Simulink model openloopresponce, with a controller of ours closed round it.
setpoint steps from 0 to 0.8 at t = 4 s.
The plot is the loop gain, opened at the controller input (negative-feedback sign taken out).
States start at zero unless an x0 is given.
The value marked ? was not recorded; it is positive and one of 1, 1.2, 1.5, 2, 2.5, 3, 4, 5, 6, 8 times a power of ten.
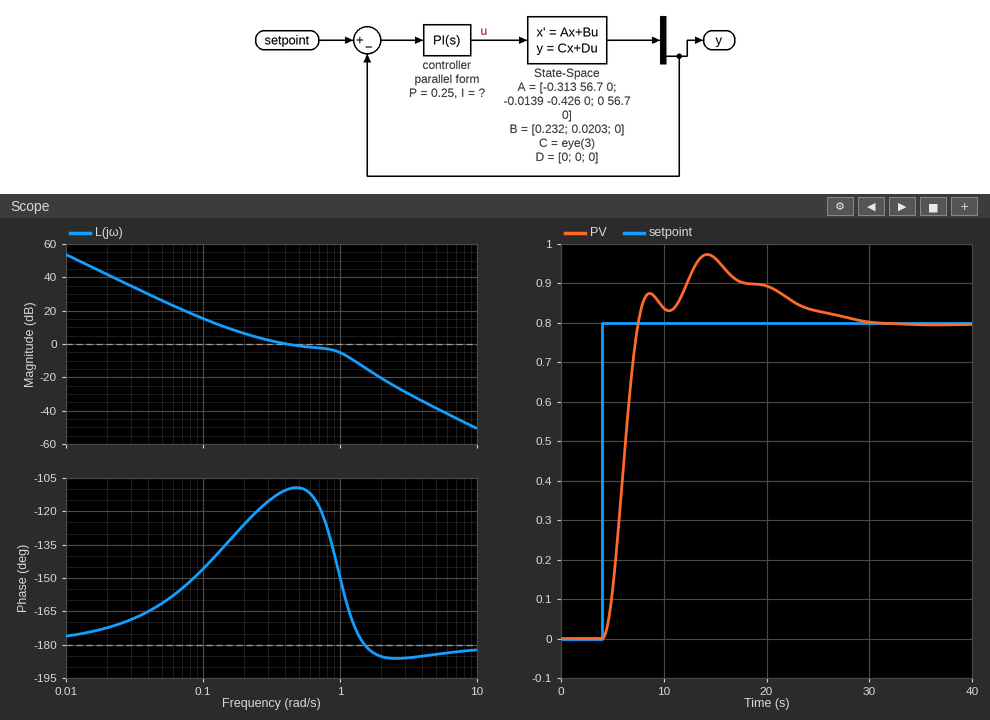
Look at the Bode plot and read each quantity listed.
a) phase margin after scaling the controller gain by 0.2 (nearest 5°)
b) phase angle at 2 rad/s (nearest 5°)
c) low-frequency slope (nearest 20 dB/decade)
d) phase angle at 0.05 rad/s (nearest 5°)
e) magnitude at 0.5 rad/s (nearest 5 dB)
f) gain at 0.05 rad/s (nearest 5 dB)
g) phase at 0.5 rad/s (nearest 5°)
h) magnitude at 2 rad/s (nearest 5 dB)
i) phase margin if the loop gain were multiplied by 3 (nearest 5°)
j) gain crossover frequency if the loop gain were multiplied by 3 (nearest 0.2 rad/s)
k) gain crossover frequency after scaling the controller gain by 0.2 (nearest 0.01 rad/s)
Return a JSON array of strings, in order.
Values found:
["35°", "-185°", "-40 dB/decade", "-160°", "0 dB", "25 dB", "-110°", "-20 dB", "10°", "1.2 rad/s", "0.11 rad/s"]
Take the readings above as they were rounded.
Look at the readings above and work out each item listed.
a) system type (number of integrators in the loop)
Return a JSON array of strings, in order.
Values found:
["2"]
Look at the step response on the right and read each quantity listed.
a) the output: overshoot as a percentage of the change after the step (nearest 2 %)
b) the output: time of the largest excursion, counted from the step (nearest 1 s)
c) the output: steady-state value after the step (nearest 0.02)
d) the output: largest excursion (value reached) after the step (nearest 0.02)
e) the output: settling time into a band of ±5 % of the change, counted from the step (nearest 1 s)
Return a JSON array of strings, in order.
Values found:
["22 %", "10 s", "0.80", "0.98", "20 s"]
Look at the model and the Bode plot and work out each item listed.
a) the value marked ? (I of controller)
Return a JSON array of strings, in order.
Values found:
["0.25"]
